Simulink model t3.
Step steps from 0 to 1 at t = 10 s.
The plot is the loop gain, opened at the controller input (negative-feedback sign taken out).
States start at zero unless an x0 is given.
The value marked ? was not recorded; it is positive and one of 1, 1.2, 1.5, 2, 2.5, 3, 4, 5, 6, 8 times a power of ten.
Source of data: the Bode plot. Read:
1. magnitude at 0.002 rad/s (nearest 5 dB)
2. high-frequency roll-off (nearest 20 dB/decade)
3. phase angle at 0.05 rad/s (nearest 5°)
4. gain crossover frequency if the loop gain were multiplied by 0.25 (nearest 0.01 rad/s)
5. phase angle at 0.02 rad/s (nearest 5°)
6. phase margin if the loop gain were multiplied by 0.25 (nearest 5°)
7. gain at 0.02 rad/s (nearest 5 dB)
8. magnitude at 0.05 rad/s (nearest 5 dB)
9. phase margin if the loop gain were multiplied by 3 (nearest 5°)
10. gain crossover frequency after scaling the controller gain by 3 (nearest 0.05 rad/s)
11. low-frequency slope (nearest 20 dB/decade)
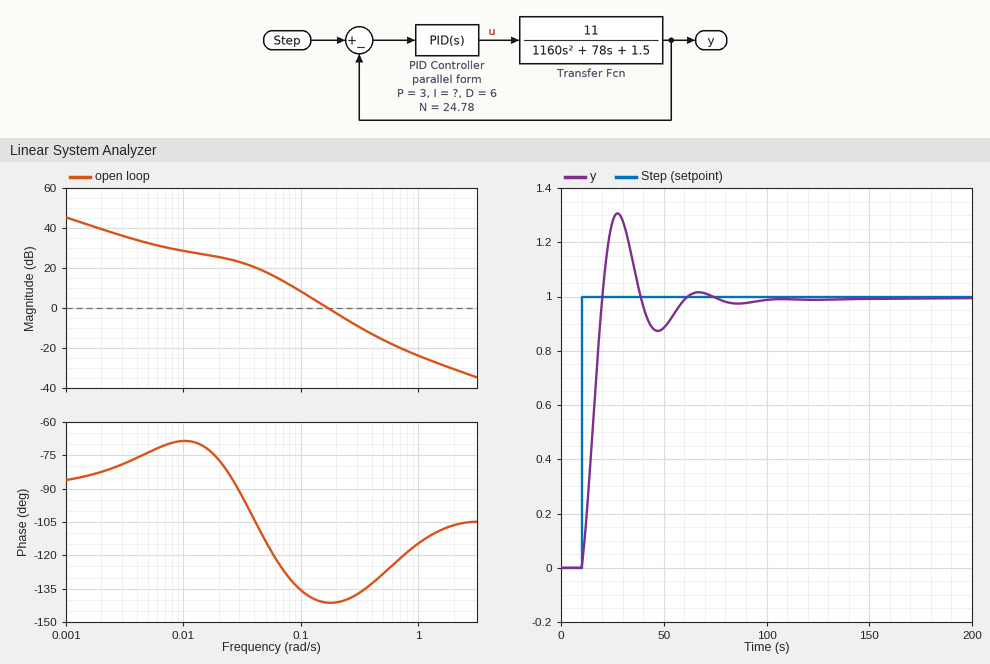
40 dB
-20 dB/decade
-115°
0.08 rad/s
-75°
50°
25 dB
20 dB
45°
0.30 rad/s
-20 dB/decade
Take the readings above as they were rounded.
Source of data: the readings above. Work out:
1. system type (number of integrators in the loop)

1
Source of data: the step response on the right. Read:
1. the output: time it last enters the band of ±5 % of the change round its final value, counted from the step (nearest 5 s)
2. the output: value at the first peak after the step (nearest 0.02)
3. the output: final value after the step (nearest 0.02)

45 s
1.30
1.00
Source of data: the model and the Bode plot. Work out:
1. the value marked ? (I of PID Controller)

0.025
